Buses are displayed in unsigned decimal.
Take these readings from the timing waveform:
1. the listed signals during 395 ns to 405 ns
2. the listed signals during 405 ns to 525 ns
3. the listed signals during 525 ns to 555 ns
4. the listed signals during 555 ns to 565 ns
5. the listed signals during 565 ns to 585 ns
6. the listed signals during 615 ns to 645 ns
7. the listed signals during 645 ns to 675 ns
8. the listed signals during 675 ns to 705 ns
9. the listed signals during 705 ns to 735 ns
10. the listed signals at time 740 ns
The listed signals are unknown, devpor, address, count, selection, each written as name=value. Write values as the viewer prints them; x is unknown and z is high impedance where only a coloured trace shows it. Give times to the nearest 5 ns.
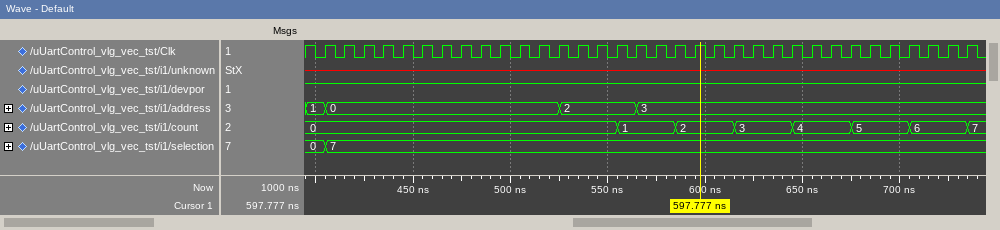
unknown=x, devpor=1, address=1, count=0, selection=0
unknown=x, devpor=1, address=0, count=0, selection=7
unknown=x, devpor=1, address=2, count=0, selection=7
unknown=x, devpor=1, address=2, count=1, selection=7
unknown=x, devpor=1, address=3, count=1, selection=7
unknown=x, devpor=1, address=3, count=3, selection=7
unknown=x, devpor=1, address=3, count=4, selection=7
unknown=x, devpor=1, address=3, count=5, selection=7
unknown=x, devpor=1, address=3, count=6, selection=7
unknown=x, devpor=1, address=3, count=7, selection=7
